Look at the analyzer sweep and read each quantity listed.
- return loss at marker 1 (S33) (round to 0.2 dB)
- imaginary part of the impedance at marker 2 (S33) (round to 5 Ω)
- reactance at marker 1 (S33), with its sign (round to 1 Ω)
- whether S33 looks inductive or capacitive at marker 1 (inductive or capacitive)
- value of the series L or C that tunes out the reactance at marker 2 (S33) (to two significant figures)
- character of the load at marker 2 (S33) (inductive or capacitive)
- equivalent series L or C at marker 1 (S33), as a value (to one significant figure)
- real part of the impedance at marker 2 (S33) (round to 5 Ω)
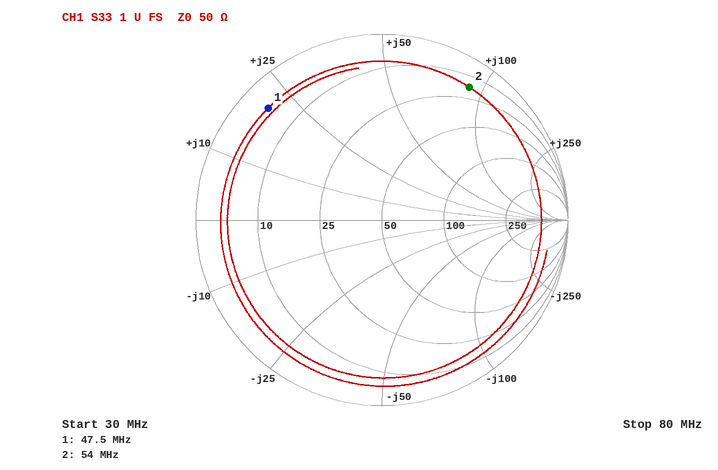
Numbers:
1.4 dB
+90 Ω
+20 Ω
inductive
33 pF
inductive
70 nH
15 Ω
